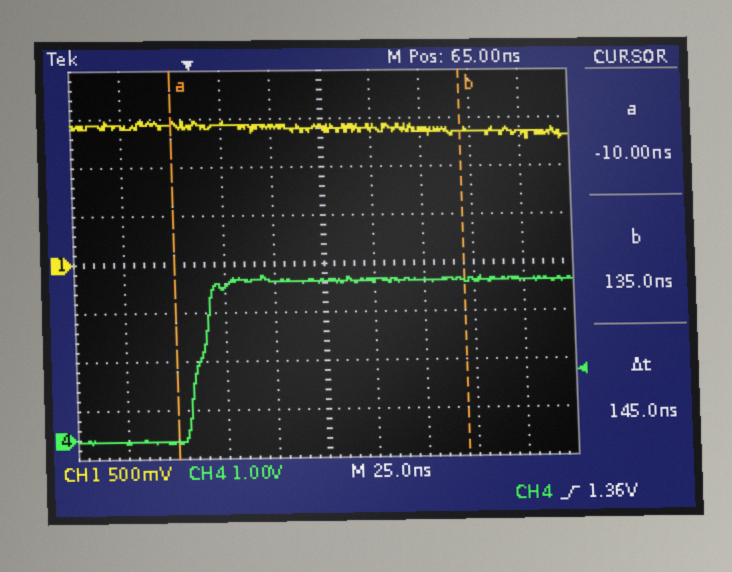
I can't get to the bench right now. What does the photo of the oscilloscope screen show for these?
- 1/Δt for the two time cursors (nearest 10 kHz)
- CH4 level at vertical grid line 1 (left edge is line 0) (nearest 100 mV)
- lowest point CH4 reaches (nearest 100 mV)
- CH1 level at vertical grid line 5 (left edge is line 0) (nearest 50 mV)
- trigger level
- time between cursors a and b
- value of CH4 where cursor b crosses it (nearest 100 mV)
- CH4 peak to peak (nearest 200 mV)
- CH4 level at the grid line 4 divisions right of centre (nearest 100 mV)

6.90 MHz
-100 mV
-100 mV
1.40 V
1.36 V
145 ns
3.2 V
3.4 V
3.2 V
